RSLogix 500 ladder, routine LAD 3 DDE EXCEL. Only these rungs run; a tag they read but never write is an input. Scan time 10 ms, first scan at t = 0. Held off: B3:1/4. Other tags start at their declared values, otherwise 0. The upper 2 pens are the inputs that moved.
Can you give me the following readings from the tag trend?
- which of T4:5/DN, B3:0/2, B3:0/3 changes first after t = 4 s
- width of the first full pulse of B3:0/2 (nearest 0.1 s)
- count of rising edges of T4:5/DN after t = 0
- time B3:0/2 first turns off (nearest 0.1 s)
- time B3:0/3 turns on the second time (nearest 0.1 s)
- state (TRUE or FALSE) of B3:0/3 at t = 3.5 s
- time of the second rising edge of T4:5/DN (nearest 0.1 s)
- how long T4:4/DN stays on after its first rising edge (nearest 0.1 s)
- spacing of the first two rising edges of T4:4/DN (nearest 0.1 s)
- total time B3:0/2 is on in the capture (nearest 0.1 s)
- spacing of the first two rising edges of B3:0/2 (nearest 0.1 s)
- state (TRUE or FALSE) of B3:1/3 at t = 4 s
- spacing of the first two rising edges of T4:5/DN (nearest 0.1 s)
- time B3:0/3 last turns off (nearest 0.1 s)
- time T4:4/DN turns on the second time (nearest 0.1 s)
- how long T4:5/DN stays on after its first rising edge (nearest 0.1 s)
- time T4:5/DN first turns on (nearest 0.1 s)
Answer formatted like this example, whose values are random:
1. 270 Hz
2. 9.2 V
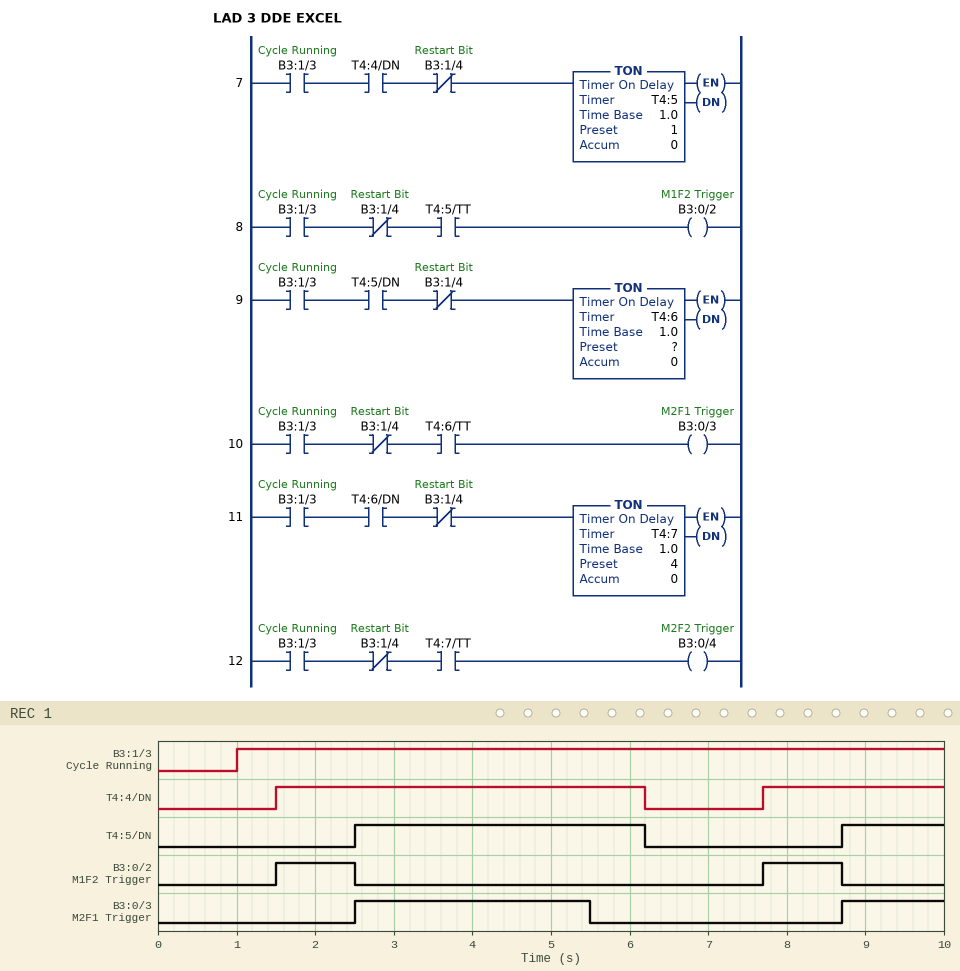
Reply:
1. B3:0/3
2. 1.0 s
3. 2
4. 2.5 s
5. 8.7 s
6. TRUE
7. 8.7 s
8. 4.7 s
9. 6.2 s
10. 2.0 s
11. 6.2 s
12. TRUE
13. 6.2 s
14. 5.5 s
15. 7.7 s
16. 3.7 s
17. 2.5 s
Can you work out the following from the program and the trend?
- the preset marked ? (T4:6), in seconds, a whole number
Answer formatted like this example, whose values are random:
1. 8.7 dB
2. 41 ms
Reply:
1. 3 s
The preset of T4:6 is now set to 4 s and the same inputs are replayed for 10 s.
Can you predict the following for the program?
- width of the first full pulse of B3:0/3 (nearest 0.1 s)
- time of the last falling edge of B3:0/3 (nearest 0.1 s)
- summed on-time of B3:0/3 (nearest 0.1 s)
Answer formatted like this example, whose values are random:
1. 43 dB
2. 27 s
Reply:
1. 3.7 s
2. 6.2 s
3. 5.0 s
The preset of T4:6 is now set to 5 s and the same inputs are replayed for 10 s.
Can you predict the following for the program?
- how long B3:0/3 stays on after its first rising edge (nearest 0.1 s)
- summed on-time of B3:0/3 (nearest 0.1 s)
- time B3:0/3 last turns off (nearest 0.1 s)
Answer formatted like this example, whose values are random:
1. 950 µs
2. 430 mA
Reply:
1. 3.7 s
2. 5.0 s
3. 6.2 s
